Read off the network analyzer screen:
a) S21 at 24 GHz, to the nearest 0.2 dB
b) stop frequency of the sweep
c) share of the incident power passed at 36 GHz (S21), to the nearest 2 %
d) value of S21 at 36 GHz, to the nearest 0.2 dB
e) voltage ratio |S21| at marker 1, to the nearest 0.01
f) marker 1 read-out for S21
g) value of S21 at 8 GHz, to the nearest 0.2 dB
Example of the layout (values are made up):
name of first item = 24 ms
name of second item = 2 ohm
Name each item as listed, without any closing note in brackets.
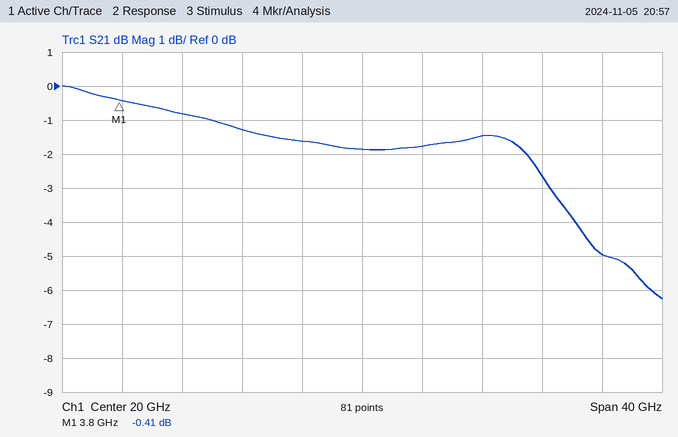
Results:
S21 at 24 GHz, to the nearest 0.2 dB = -1.8 dB
stop frequency of the sweep = 40 GHz
share of the incident power passed at 36 GHz (S21), to the nearest 2 % = 32 %
value of S21 at 36 GHz, to the nearest 0.2 dB = -5.0 dB
voltage ratio |S21| at marker 1, to the nearest 0.01 = 0.95
marker 1 read-out for S21 = -0.41 dB
value of S21 at 8 GHz, to the nearest 0.2 dB = -0.8 dB
